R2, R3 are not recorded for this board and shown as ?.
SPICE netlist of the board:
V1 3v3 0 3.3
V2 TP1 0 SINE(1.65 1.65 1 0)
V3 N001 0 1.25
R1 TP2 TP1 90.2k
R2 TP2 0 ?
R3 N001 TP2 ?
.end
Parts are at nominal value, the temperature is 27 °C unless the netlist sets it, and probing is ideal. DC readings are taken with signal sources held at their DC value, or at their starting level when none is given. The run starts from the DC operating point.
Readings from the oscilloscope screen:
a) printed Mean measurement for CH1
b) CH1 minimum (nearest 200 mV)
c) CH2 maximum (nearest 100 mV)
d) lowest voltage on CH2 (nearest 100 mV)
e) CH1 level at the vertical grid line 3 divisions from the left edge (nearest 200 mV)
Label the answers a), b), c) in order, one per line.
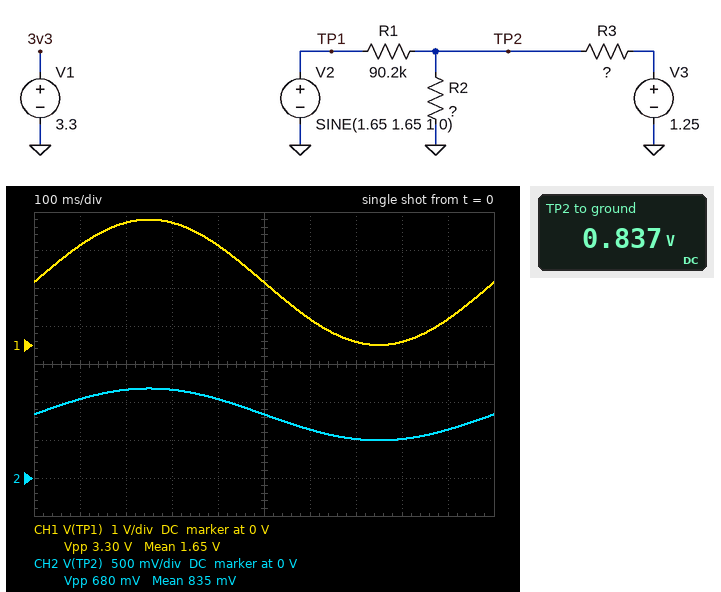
a) 1.65 V
b) 0 V
c) 1.2 V
d) 500 mV
e) 3.2 V
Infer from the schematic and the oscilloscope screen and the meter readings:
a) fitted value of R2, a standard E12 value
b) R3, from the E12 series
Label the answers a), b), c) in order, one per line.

a) 47 kΩ
b) 47 kΩ
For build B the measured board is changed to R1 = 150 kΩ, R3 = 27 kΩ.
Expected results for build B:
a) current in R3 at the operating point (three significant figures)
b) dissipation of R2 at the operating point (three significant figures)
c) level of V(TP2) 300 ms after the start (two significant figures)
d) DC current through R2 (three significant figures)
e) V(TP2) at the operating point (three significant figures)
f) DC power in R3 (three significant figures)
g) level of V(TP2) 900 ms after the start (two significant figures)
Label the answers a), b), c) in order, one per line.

a) 13.6 µA
b) 16.5 µW
c) 1.0 V
d) 18.8 µA
e) 882 mV
f) 5.02 µW
g) 780 mV
